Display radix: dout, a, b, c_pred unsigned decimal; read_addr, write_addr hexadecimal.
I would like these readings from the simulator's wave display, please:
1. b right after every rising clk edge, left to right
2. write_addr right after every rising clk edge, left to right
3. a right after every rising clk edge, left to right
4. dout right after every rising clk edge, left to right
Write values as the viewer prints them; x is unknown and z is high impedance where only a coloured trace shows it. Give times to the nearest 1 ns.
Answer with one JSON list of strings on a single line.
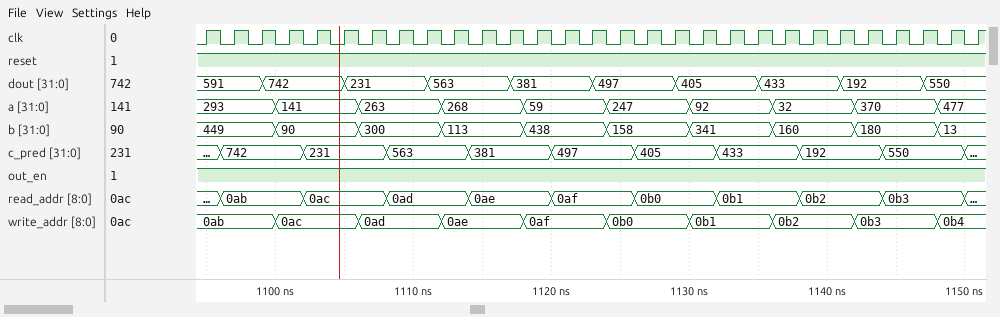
["449, 449, 449, 90, 90, 90, 300, 300, 300, 113, 113, 113, 438, 438, 438, 158, 158, 158, 341, 341, 341, 160, 160, 160, 180, 180, 180, 13, 13", "0ab, 0ab, 0ab, 0ac, 0ac, 0ac, 0ad, 0ad, 0ad, 0ae, 0ae, 0ae, 0af, 0af, 0af, 0b0, 0b0, 0b0, 0b1, 0b1, 0b1, 0b2, 0b2, 0b2, 0b3, 0b3, 0b3, 0b4, 0b4", "293, 293, 293, 141, 141, 141, 263, 263, 263, 268, 268, 268, 59, 59, 59, 247, 247, 247, 92, 92, 92, 32, 32, 32, 370, 370, 370, 477, 477", "591, 591, 742, 742, 742, 231, 231, 231, 563, 563, 563, 381, 381, 381, 497, 497, 497, 405, 405, 405, 433, 433, 433, 192, 192, 192, 550, 550, 550"]
